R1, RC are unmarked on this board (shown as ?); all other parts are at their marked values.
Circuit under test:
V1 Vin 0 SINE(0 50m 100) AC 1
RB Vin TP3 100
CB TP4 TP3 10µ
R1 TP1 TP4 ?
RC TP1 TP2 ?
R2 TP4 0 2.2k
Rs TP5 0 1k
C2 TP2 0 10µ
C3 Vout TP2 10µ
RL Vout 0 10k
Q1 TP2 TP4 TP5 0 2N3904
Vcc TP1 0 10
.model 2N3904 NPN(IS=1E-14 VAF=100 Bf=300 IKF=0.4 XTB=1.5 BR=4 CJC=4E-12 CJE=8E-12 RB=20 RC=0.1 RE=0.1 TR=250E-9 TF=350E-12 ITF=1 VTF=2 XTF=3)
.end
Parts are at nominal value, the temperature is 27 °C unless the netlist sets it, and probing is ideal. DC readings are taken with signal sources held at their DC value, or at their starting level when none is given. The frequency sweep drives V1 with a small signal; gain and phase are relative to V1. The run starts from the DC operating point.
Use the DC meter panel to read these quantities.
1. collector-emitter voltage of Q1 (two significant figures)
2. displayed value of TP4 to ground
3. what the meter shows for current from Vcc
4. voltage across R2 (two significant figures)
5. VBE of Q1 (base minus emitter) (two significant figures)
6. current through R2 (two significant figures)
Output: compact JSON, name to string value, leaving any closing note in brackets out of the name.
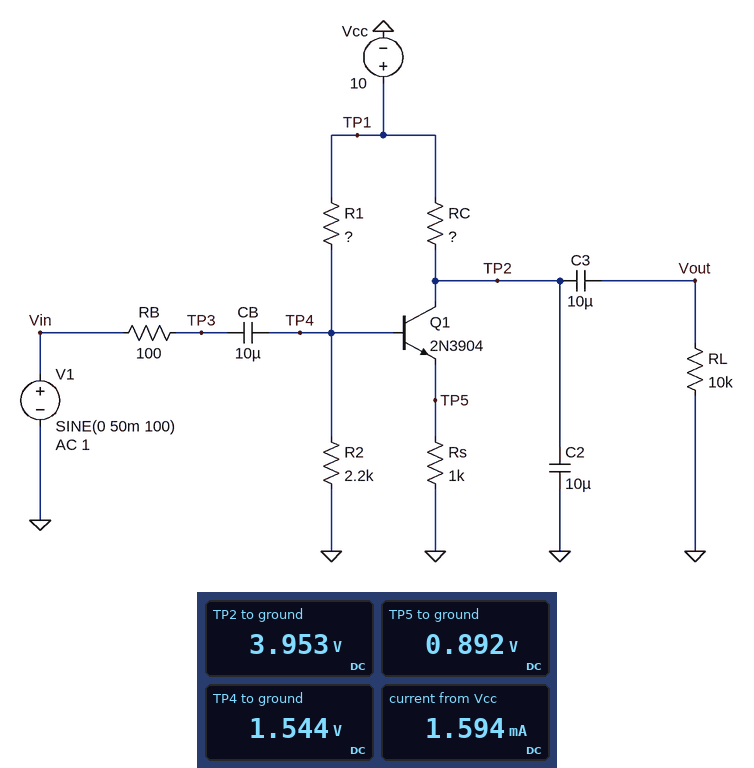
{"collector-emitter voltage of Q1": "3.1 V", "displayed value of TP4 to ground": "1.544 V", "what the meter shows for current from Vcc": "1.594 mA", "voltage across R2": "1.5 V", "VBE of Q1 (base minus emitter)": "650 mV", "current through R2": "700 µA"}
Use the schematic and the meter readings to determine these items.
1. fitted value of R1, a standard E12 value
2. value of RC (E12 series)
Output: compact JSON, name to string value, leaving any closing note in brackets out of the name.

{"fitted value of R1, a standard E12 value": "12 kΩ", "value of RC": "6.8 kΩ"}
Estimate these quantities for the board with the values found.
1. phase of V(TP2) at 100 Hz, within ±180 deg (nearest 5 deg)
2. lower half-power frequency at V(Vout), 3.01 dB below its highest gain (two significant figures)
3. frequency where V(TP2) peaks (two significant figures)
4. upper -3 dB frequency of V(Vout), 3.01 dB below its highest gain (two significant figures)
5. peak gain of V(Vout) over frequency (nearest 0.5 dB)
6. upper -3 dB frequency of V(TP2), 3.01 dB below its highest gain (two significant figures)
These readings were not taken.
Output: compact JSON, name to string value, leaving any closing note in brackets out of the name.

{"phase of V(TP2) at 100 Hz, within ±180 deg": "95 deg", "lower half-power frequency at V(Vout), 3.01 dB below its highest gain": "2.6 Hz", "frequency where V(TP2) peaks": "5.9 Hz", "upper -3 dB frequency of V(Vout), 3.01 dB below its highest gain": "16 Hz", "peak gain of V(Vout) over frequency": "1.0 dB", "upper -3 dB frequency of V(TP2), 3.01 dB below its highest gain": "15 Hz"}
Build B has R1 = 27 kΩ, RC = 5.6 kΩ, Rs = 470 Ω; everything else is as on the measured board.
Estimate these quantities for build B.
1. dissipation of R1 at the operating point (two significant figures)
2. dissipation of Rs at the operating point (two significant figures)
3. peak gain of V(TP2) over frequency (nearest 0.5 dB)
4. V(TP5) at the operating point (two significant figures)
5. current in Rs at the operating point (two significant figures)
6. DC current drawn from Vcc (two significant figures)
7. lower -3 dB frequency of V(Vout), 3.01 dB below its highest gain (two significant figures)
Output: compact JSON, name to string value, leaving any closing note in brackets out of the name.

{"dissipation of R1 at the operating point": "3.2 mW", "dissipation of Rs at the operating point": "37 µW", "peak gain of V(TP2) over frequency": "6.5 dB", "V(TP5) at the operating point": "130 mV", "current in Rs at the operating point": "280 µA", "DC current drawn from Vcc": "620 µA", "lower -3 dB frequency of V(Vout), 3.01 dB below its highest gain": "2.7 Hz"}
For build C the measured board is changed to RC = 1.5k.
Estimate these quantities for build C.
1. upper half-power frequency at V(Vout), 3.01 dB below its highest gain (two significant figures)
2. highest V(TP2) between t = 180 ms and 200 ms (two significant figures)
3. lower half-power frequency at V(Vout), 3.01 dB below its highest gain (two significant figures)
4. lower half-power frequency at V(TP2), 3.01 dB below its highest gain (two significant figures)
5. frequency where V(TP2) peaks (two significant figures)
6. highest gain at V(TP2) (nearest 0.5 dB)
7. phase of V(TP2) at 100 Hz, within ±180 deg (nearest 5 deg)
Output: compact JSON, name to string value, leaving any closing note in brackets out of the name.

{"upper half-power frequency at V(Vout), 3.01 dB below its highest gain": "25 Hz", "highest V(TP2) between t = 180 ms and 200 ms": "8.7 V", "lower half-power frequency at V(Vout), 3.01 dB below its highest gain": "4.3 Hz", "lower half-power frequency at V(TP2), 3.01 dB below its highest gain": "4.0 Hz", "frequency where V(TP2) peaks": "10 Hz", "highest gain at V(TP2)": "-3.0 dB", "phase of V(TP2) at 100 Hz, within ±180 deg": "100 deg"}
